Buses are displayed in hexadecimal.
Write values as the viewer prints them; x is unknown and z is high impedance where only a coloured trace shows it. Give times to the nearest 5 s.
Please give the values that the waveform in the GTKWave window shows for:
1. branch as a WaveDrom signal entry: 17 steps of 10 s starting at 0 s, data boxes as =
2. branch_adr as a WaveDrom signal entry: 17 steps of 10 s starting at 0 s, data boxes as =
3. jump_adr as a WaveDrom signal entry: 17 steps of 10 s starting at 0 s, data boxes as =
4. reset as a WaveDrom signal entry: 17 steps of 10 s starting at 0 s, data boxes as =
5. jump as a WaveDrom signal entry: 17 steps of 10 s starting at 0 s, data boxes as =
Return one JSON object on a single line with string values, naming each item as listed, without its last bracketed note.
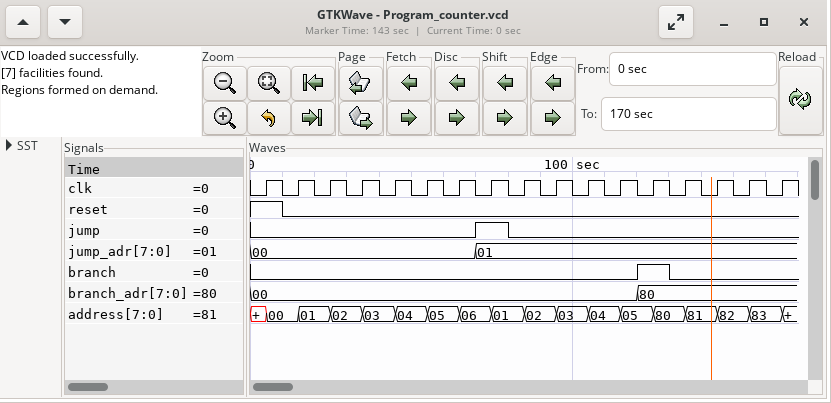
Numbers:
{"branch as a WaveDrom signal entry: 17 steps of 10 s starting at 0 s, data boxes as =": "{name: 'branch', wave: '0...........10...'}", "branch_adr as a WaveDrom signal entry: 17 steps of 10 s starting at 0 s, data boxes as =": "{name: 'branch_adr', wave: '=...........=....', data: '00 80'}", "jump_adr as a WaveDrom signal entry: 17 steps of 10 s starting at 0 s, data boxes as =": "{name: 'jump_adr', wave: '=......=.........', data: '00 01'}", "reset as a WaveDrom signal entry: 17 steps of 10 s starting at 0 s, data boxes as =": "{name: 'reset', wave: '10...............'}", "jump as a WaveDrom signal entry: 17 steps of 10 s starting at 0 s, data boxes as =": "{name: 'jump', wave: '0......10........'}"}
